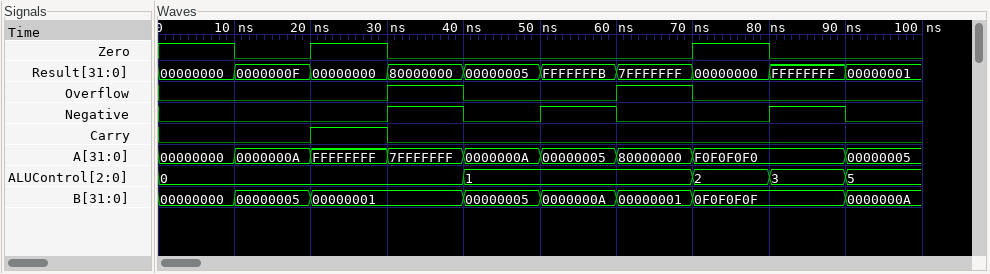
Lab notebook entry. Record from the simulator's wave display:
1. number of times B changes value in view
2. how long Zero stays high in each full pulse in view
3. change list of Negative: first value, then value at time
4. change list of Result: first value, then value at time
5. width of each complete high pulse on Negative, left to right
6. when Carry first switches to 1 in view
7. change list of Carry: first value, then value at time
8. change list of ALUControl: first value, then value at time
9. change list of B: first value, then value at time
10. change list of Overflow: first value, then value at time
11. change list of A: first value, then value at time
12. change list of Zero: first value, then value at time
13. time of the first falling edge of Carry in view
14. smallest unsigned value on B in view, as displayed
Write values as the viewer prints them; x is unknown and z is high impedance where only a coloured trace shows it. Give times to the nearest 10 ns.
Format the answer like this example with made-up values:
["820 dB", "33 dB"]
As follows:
["7", "10 ns, 10 ns", "0, 1 at 30 ns, 0 at 40 ns, 1 at 50 ns, 0 at 60 ns, 1 at 80 ns, 0 at 90 ns", "00000000, 0000000F at 10 ns, 00000000 at 20 ns, 80000000 at 30 ns, 00000005 at 40 ns, FFFFFFFB at 50 ns, 7FFFFFFF at 60 ns, 00000000 at 70 ns, FFFFFFFF at 80 ns, 00000001 at 90 ns", "10 ns, 10 ns, 10 ns", "20 ns", "0, 1 at 20 ns, 0 at 30 ns", "0, 1 at 40 ns, 2 at 70 ns, 3 at 80 ns, 5 at 90 ns", "00000000, 00000005 at 10 ns, 00000001 at 20 ns, 00000005 at 40 ns, 0000000A at 50 ns, 00000001 at 60 ns, 0F0F0F0F at 70 ns, 0000000A at 90 ns", "0, 1 at 30 ns, 0 at 40 ns, 1 at 60 ns, 0 at 70 ns", "00000000, 0000000A at 10 ns, FFFFFFFF at 20 ns, 7FFFFFFF at 30 ns, 0000000A at 40 ns, 00000005 at 50 ns, 80000000 at 60 ns, F0F0F0F0 at 70 ns, 00000005 at 90 ns", "1, 0 at 10 ns, 1 at 20 ns, 0 at 30 ns, 1 at 70 ns, 0 at 80 ns", "30 ns", "00000000"]
